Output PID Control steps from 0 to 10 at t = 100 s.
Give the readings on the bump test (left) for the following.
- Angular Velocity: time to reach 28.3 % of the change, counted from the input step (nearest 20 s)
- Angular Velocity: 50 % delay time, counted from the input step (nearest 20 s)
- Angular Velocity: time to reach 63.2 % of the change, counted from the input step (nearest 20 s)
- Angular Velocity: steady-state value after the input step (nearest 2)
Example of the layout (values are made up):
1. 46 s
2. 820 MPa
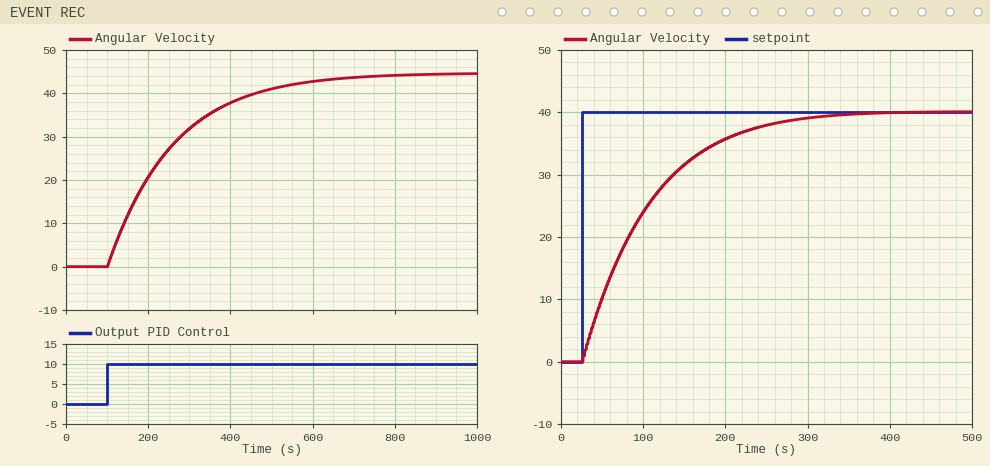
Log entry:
1. 60 s
2. 120 s
3. 160 s
4. 44
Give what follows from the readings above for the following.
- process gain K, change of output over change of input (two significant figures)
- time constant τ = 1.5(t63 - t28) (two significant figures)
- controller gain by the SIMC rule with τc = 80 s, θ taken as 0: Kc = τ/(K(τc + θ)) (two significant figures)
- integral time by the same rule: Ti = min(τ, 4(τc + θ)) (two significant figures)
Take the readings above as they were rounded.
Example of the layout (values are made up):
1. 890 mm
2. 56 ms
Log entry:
1. 4.4
2. 150 s
3. 0.43
4. 150 s
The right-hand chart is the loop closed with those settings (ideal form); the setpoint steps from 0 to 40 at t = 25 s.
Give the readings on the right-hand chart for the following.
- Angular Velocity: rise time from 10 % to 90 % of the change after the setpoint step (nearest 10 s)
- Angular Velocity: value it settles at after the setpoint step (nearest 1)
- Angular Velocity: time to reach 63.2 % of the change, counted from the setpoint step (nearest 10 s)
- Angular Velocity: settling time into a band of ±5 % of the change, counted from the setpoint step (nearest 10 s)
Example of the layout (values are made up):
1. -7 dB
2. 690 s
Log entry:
1. 170 s
2. 40
3. 80 s
4. 230 s
